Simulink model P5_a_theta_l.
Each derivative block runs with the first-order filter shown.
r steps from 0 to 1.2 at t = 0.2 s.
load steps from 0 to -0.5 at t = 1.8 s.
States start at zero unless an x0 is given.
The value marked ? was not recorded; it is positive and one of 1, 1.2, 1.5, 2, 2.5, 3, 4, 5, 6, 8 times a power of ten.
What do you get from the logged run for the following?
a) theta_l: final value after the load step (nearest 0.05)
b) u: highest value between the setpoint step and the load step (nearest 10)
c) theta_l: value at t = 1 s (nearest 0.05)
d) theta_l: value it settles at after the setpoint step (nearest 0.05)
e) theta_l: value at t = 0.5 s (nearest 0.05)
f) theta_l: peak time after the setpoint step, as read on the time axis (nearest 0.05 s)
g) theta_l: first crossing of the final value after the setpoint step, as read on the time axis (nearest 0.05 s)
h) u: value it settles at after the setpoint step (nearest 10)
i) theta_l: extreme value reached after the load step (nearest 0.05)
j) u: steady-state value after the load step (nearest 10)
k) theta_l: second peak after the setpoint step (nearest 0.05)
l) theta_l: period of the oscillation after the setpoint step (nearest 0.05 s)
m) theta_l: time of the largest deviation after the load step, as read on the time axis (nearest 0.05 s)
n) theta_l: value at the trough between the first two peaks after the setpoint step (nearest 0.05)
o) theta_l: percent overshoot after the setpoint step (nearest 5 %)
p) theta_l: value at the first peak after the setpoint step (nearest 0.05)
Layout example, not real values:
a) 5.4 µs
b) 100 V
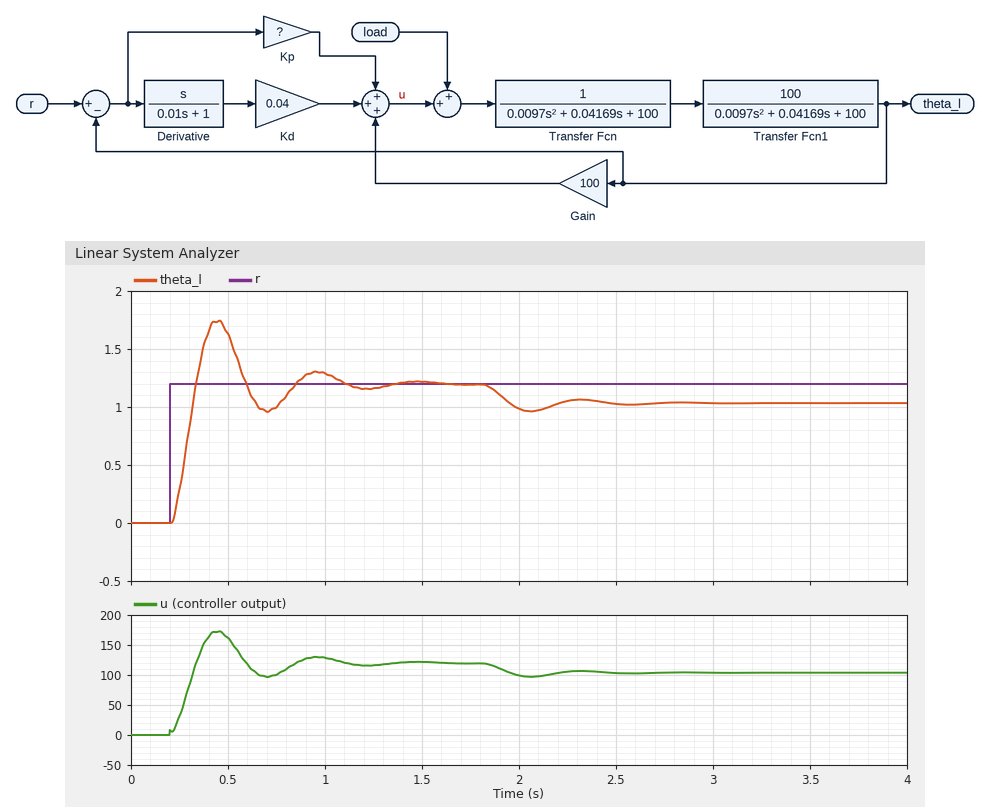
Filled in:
a) 1.05
b) 170
c) 1.30
d) 1.20
e) 1.65
f) 0.45 s
g) 0.35 s
h) 120
i) 0.95
j) 100
k) 1.30
l) 0.50 s
m) 2.05 s
n) 0.95
o) 45 %
p) 1.75
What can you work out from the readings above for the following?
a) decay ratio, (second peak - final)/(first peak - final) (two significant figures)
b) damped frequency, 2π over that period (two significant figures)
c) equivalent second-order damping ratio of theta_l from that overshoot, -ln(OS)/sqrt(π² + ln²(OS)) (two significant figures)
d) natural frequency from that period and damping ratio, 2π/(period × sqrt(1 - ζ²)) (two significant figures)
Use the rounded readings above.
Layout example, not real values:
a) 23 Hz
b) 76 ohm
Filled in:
a) 0.18
b) 13 rad/s
c) 0.25
d) 13 rad/s
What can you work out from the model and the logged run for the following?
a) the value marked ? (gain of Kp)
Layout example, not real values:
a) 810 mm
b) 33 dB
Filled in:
a) 3
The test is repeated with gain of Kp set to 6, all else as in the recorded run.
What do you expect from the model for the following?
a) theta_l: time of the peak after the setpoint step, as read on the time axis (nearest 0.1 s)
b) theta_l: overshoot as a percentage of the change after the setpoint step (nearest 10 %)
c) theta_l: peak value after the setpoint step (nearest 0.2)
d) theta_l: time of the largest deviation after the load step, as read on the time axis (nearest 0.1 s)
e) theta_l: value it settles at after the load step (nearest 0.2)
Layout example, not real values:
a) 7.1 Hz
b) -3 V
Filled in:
a) 0.4 s
b) 60 %
c) 2.0
d) 2.0 s
e) 1.2
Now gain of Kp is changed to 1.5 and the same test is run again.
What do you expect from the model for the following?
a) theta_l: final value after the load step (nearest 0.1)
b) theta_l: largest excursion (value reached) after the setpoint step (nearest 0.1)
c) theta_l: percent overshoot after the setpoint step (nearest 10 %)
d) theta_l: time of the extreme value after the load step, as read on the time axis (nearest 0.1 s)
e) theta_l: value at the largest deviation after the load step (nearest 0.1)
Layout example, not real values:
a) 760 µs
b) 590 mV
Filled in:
a) 0.9
b) 1.6
c) 30 %
d) 2.2 s
e) 0.8
